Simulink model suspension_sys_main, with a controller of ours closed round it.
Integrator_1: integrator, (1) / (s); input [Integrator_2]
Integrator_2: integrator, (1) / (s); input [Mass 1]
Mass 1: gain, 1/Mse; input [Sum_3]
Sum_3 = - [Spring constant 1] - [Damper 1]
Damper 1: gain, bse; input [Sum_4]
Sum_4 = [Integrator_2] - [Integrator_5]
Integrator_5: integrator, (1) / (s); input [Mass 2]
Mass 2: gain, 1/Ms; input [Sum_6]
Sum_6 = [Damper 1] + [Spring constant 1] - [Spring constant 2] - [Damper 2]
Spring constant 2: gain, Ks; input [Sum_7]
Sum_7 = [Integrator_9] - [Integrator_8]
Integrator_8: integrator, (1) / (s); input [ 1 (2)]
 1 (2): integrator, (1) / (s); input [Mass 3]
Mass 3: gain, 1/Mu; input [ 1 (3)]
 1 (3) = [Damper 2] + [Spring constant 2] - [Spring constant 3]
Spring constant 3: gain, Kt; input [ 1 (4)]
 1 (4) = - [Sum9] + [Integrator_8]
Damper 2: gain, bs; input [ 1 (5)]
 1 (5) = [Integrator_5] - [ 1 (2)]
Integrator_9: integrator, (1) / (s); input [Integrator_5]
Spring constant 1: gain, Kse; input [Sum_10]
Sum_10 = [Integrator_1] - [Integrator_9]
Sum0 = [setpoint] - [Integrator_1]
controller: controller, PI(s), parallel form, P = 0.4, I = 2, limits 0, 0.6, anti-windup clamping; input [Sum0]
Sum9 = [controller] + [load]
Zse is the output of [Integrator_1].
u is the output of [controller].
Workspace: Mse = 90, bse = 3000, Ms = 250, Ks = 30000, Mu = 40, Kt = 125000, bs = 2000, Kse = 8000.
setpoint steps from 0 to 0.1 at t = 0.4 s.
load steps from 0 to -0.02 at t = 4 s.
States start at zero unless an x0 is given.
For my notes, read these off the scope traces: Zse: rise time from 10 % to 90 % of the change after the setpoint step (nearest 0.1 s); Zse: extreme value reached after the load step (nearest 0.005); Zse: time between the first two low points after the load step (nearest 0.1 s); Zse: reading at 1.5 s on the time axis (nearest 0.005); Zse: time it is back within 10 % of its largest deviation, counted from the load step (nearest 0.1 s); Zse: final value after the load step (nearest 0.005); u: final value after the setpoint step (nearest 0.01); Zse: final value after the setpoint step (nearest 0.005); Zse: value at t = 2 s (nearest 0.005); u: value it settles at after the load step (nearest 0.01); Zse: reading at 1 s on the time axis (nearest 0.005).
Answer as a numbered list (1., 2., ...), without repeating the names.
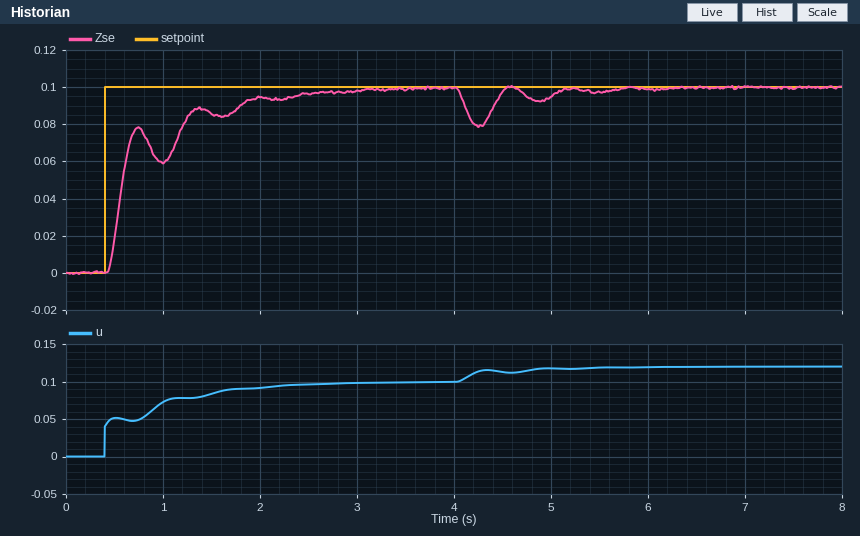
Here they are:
1. 1.3 s
2. 0.080
3. 0.6 s
4. 0.085
5. 1.6 s
6. 0.100
7. 0.10
8. 0.100
9. 0.095
10. 0.12
11. 0.060
